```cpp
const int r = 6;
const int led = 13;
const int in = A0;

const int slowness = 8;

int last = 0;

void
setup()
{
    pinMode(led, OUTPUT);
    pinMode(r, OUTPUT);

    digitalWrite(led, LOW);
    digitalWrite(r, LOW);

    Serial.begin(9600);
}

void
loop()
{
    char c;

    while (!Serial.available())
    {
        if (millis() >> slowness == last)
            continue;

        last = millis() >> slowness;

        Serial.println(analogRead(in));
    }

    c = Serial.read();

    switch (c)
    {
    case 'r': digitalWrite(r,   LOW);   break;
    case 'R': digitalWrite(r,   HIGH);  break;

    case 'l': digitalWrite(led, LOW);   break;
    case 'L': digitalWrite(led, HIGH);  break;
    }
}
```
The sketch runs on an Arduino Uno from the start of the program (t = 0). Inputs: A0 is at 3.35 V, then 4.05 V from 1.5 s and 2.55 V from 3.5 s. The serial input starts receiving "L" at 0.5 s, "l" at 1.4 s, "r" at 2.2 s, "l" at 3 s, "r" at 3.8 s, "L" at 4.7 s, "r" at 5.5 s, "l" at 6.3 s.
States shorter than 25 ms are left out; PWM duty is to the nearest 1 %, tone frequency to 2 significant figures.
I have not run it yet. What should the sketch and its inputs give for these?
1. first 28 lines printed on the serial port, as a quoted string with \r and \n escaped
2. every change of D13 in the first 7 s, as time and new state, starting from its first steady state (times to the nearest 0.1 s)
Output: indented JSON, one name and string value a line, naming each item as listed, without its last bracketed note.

{
  "first 28 lines printed on the serial port, as a quoted string with \\r and \\n escaped": "\"686\\r\\n686\\r\\n686\\r\\n686\\r\\n686\\r\\n829\\r\\n829\\r\\n829\\r\\n829\\r\\n829\\r\\n829\\r\\n829\\r\\n829\\r\\n522\\r\\n522\\r\\n522\\r\\n522\\r\\n522\\r\\n522\\r\\n522\\r\\n522\\r\\n522\\r\\n522\\r\\n522\\r\\n522\\r\\n522\\r\\n522\\r\\n522\\r\\n\"",
  "every change of D13 in the first 7 s, as time and new state, starting from its first steady state": "0 s low; 0.5 s high; 1.4 s low; 4.7 s high; 6.3 s low"
}
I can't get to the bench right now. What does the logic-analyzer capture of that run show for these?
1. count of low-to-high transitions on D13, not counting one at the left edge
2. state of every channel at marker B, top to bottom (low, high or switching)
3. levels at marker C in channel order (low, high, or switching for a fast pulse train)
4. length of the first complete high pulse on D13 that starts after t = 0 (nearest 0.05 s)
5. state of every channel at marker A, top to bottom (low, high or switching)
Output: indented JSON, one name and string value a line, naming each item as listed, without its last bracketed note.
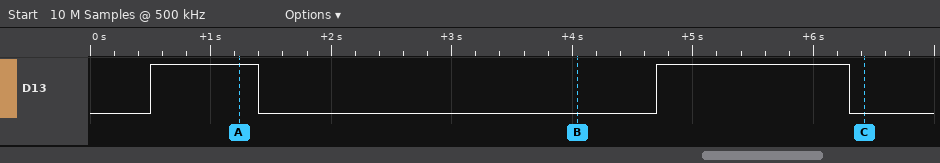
{
  "count of low-to-high transitions on D13, not counting one at the left edge": "2",
  "state of every channel at marker B, top to bottom": "D13 low",
  "levels at marker C in channel order": "D13 low",
  "length of the first complete high pulse on D13 that starts after t = 0": "0.90 s",
  "state of every channel at marker A, top to bottom": "D13 high"
}
